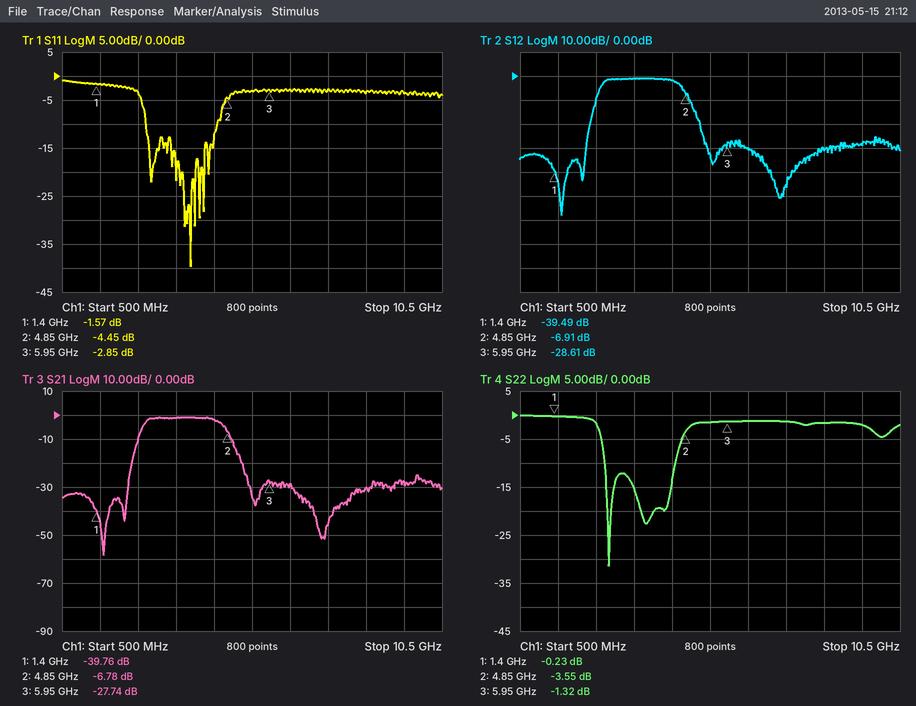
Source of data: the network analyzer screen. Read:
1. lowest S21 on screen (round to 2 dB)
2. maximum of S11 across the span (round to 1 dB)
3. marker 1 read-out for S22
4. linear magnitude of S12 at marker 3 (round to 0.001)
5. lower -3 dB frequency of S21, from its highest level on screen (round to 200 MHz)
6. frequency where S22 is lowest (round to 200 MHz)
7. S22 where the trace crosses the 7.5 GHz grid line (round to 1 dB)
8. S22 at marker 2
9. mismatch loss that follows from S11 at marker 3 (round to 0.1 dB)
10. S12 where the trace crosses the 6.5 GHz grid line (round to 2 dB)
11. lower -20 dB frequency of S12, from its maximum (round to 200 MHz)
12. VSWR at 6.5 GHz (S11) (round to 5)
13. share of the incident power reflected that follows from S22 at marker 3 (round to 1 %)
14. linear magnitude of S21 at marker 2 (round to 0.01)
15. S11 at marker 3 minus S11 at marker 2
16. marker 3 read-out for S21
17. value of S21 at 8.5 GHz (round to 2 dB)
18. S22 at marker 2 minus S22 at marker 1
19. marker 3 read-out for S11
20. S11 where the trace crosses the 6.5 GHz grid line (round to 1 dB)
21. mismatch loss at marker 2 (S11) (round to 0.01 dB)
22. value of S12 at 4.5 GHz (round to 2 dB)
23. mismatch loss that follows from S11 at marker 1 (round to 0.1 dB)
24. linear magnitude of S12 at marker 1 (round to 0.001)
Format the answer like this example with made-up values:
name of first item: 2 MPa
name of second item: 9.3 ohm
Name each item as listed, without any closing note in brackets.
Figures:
lowest S21 on screen: -58 dB
maximum of S11 across the span: -1 dB
marker 1 read-out for S22: -0.23 dB
linear magnitude of S12 at marker 3: 0.037
lower -3 dB frequency of S21, from its highest level on screen: 2.6 GHz
frequency where S22 is lowest: 2.8 GHz
S22 where the trace crosses the 7.5 GHz grid line: -1 dB
S22 at marker 2: -3.55 dB
mismatch loss that follows from S11 at marker 3: 3.2 dB
S12 where the trace crosses the 6.5 GHz grid line: -30 dB
lower -20 dB frequency of S12, from its maximum: 2.4 GHz
VSWR at 6.5 GHz (S11): 5
share of the incident power reflected that follows from S22 at marker 3: 74 %
linear magnitude of S21 at marker 2: 0.46
S11 at marker 3 minus S11 at marker 2: 1.60 dB
marker 3 read-out for S21: -27.74 dB
value of S21 at 8.5 GHz: -30 dB
S22 at marker 2 minus S22 at marker 1: -3.32 dB
marker 3 read-out for S11: -2.85 dB
S11 where the trace crosses the 6.5 GHz grid line: -3 dB
mismatch loss at marker 2 (S11): 1.93 dB
value of S12 at 4.5 GHz: -2 dB
mismatch loss that follows from S11 at marker 1: 5.2 dB
linear magnitude of S12 at marker 1: 0.011
